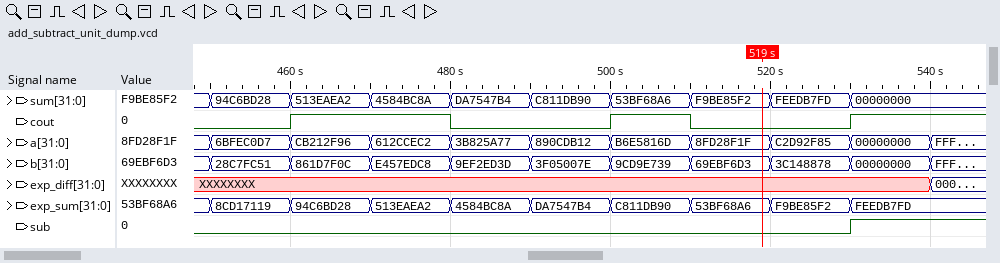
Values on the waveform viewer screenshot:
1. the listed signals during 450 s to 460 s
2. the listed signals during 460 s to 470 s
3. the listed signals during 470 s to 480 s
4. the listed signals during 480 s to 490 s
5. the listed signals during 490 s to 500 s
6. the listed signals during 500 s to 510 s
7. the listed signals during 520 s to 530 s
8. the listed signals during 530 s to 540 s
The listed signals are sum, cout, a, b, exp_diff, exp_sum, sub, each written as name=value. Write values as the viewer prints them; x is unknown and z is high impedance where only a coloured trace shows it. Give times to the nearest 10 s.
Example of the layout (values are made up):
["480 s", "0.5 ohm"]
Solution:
["sum=94C6BD28, cout=0, a=6BFEC0D7, b=28C7FC51, exp_diff=XXXXXXXX, exp_sum=8CD17119, sub=0", "sum=513EAEA2, cout=1, a=CB212F96, b=861D7F0C, exp_diff=XXXXXXXX, exp_sum=94C6BD28, sub=0", "sum=4584BC8A, cout=1, a=612CCEC2, b=E457EDC8, exp_diff=XXXXXXXX, exp_sum=513EAEA2, sub=0", "sum=DA7547B4, cout=0, a=3B825A77, b=9EF2ED3D, exp_diff=XXXXXXXX, exp_sum=4584BC8A, sub=0", "sum=C811DB90, cout=0, a=890CDB12, b=3F05007E, exp_diff=XXXXXXXX, exp_sum=DA7547B4, sub=0", "sum=53BF68A6, cout=1, a=B6E5816D, b=9CD9E739, exp_diff=XXXXXXXX, exp_sum=C811DB90, sub=0", "sum=FEEDB7FD, cout=0, a=C2D92F85, b=3C148878, exp_diff=XXXXXXXX, exp_sum=F9BE85F2, sub=0", "sum=00000000, cout=1, a=00000000, b=00000000, exp_diff=XXXXXXXX, exp_sum=FEEDB7FD, sub=1"]
